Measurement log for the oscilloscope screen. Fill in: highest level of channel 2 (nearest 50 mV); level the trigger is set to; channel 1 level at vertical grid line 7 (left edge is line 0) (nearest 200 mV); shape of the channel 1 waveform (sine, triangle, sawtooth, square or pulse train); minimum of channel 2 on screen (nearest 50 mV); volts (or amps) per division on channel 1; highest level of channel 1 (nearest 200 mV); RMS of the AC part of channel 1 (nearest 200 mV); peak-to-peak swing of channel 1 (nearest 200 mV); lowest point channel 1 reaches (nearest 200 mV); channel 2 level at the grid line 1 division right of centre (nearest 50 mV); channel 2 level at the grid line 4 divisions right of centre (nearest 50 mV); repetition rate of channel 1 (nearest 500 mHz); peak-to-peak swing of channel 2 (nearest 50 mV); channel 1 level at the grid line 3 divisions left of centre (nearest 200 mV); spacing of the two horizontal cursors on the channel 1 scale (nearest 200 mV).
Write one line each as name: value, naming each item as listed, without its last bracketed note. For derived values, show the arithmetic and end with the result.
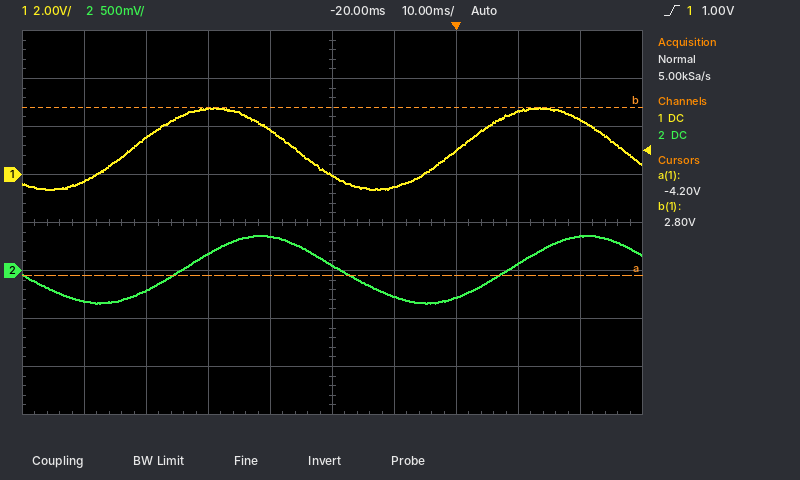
highest level of channel 2: 350 mV
level the trigger is set to: 1.00 V
channel 1 level at vertical grid line 7 (left edge is line 0): 1.0 V
shape of the channel 1 waveform: sine
minimum of channel 2 on screen: -350 mV
volts (or amps) per division on channel 1: 2 V
highest level of channel 1: 2.8 V
RMS of the AC part of channel 1: 3.4 V / (2√2) ≈ 1.2 V
peak-to-peak swing of channel 1: 2.8 V − (-600 mV) = 3.4 V
lowest point channel 1 reaches: -600 mV
channel 2 level at the grid line 1 division right of centre: -250 mV
channel 2 level at the grid line 4 divisions right of centre: 350 mV
repetition rate of channel 1: 19.0 Hz
peak-to-peak swing of channel 2: 350 mV − (-350 mV) = 700 mV
channel 1 level at the grid line 3 divisions left of centre: 1.6 V
spacing of the two horizontal cursors on the channel 1 scale: 7.0 V
